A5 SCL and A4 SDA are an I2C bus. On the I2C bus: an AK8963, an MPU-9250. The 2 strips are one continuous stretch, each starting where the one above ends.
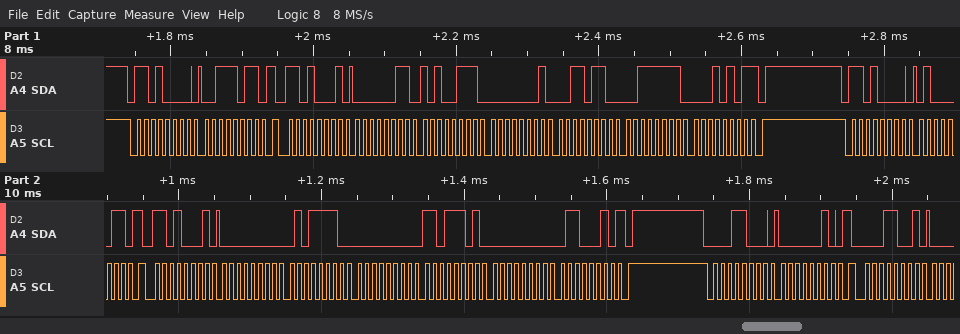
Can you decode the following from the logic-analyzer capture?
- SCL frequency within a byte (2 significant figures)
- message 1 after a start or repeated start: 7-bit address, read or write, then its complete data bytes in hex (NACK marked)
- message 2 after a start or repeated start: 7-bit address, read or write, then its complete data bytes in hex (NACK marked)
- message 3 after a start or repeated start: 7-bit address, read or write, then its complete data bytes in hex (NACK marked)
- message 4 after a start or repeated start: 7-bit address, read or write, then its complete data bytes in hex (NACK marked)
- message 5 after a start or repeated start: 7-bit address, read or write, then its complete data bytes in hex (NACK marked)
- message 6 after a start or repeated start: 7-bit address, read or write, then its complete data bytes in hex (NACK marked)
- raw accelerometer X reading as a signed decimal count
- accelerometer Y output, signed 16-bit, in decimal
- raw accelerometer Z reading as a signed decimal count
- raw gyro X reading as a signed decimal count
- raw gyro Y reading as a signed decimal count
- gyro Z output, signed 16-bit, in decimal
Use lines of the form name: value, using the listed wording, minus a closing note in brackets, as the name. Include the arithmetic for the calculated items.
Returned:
SCL frequency within a byte: 100 kHz
message 1 after a start or repeated start: 7-bit address, read or write, then its complete data bytes in hex: 0x68 write: 3B
message 2 after a start or repeated start: 7-bit address, read or write, then its complete data bytes in hex: 0x68 read: 03 A7 01 36 3F 15 NACK
message 3 after a start or repeated start: 7-bit address, read or write, then its complete data bytes in hex: 0x68 write: 43
message 4 after a start or repeated start: 7-bit address, read or write, then its complete data bytes in hex: 0x68 read: 00 5E 00 DD 00 62 NACK
message 5 after a start or repeated start: 7-bit address, read or write, then its complete data bytes in hex: 0x0C write: 02
message 6 after a start or repeated start: 7-bit address, read or write, then its complete data bytes in hex: 0x0C read
raw accelerometer X reading as a signed decimal count: 0x03A7 = 935
accelerometer Y output, signed 16-bit, in decimal: 0x0136 = 310
raw accelerometer Z reading as a signed decimal count: 0x3F15 = 16149
raw gyro X reading as a signed decimal count: 0x005E = 94
raw gyro Y reading as a signed decimal count: 0x00DD = 221
gyro Z output, signed 16-bit, in decimal: 0x0062 = 98
